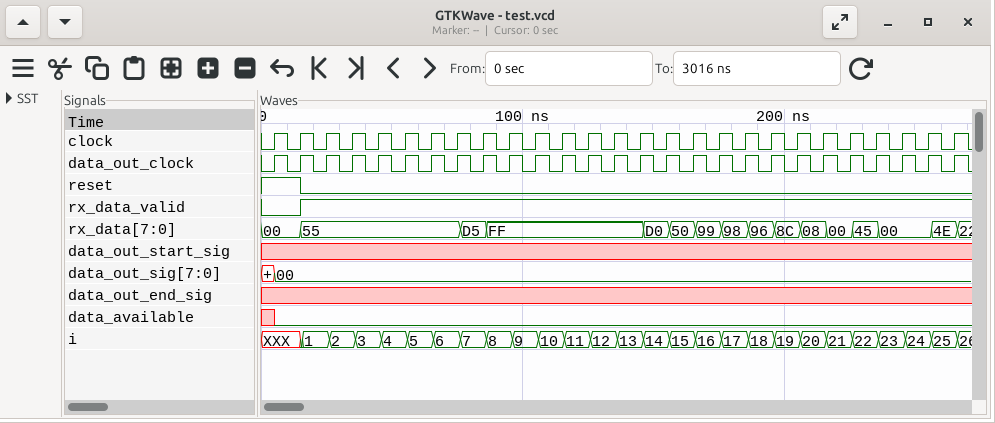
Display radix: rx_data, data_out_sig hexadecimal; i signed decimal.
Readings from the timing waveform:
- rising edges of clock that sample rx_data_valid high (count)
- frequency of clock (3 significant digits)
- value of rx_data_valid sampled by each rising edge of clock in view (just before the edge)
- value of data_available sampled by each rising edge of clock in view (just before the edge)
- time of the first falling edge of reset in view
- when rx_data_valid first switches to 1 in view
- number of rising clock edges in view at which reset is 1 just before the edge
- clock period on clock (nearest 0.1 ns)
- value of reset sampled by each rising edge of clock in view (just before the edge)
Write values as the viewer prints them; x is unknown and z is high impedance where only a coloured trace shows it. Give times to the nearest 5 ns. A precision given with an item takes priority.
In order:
25
100 MHz
0 0 1 1 1 1 1 1 1 1 1 1 1 1 1 1 1 1 1 1 1 1 1 1 1 1 1
x 0 0 0 0 0 0 0 0 0 0 0 0 0 0 0 0 0 0 0 0 0 0 0 0 0 0
15 ns
15 ns
2
10 ns
1 1 0 0 0 0 0 0 0 0 0 0 0 0 0 0 0 0 0 0 0 0 0 0 0 0 0
